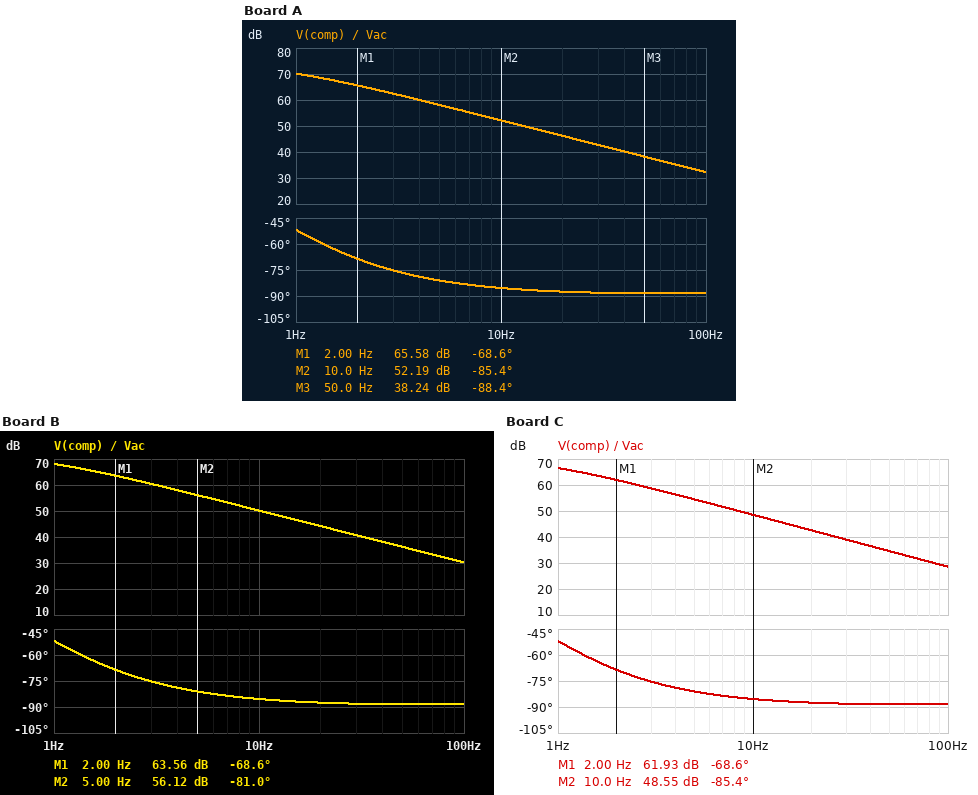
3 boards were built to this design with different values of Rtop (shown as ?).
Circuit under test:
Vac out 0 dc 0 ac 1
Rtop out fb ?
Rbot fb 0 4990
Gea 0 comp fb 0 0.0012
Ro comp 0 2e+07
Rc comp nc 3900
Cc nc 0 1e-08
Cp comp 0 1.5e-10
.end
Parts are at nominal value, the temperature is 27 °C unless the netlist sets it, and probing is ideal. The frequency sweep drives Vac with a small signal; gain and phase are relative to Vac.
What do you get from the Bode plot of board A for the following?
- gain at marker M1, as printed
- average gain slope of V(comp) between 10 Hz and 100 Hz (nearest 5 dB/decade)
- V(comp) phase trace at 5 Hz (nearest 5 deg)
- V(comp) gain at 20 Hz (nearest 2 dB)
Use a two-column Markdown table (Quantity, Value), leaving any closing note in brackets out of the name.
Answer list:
| Quantity | Value |
|---|---|
| gain at marker M1, as printed | 65.58 dB |
| average gain slope of V(comp) between 10 Hz and 100 Hz | -20 dB/decade |
| V(comp) phase trace at 5 Hz | -80 deg |
| V(comp) gain at 20 Hz | 46 dB |
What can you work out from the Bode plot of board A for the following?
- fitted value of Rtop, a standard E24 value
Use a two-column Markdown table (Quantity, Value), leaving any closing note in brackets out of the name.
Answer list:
| Quantity | Value |
|---|---|
| fitted value of Rtop, a standard E24 value | 18 kΩ |
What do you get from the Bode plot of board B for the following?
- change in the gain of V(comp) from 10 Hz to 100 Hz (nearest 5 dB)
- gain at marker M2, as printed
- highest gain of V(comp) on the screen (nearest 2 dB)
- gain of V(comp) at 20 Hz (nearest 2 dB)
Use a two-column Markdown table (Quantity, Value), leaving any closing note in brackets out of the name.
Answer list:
| Quantity | Value |
|---|---|
| change in the gain of V(comp) from 10 Hz to 100 Hz | -20 dB |
| gain at marker M2, as printed | 56.12 dB |
| highest gain of V(comp) on the screen | 68 dB |
| gain of V(comp) at 20 Hz | 44 dB |
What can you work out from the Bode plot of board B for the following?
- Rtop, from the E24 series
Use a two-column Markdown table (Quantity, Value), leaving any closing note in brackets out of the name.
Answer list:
| Quantity | Value |
|---|---|
| Rtop, from the E24 series | 24 kΩ |
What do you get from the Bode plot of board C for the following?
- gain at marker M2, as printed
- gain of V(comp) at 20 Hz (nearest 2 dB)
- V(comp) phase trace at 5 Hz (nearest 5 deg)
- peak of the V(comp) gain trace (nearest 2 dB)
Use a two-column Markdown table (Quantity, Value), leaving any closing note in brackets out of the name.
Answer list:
| Quantity | Value |
|---|---|
| gain at marker M2, as printed | 48.55 dB |
| gain of V(comp) at 20 Hz | 42 dB |
| V(comp) phase trace at 5 Hz | -80 deg |
| peak of the V(comp) gain trace | 66 dB |
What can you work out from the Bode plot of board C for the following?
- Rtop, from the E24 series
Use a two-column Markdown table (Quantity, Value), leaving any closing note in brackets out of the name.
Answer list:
| Quantity | Value |
|---|---|
| Rtop, from the E24 series | 30 kΩ |
